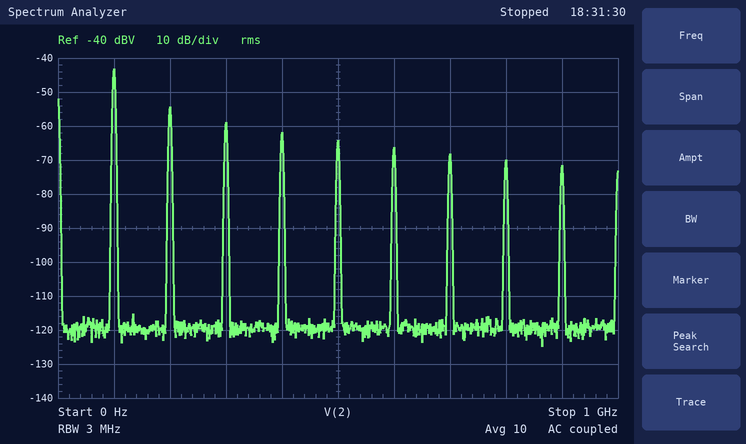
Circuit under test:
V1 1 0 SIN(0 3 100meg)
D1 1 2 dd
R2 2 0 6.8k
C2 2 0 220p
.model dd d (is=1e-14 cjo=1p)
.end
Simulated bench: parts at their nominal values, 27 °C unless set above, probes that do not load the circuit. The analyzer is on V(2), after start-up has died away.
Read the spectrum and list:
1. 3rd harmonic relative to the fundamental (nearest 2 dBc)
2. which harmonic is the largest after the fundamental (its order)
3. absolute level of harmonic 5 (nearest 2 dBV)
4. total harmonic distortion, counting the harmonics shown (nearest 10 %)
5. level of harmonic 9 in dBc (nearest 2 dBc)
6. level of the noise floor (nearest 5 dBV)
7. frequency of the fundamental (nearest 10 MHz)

-16 dBc
2
-64 dBV
40 %
-28 dBc
-120 dBV
100 MHz
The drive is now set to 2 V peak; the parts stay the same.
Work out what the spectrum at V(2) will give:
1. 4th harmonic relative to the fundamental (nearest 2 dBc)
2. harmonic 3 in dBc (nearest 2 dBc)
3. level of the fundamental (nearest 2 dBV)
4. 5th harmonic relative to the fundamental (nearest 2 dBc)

-22 dBc
-18 dBc
-46 dBV
-24 dBc
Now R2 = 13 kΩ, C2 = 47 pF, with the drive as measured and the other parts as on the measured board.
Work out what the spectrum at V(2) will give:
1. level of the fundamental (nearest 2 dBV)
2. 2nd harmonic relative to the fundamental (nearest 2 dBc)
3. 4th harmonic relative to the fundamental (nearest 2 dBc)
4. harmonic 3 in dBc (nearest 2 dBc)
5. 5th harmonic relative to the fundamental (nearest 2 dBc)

-30 dBV
-14 dBc
-24 dBc
-20 dBc
-26 dBc
